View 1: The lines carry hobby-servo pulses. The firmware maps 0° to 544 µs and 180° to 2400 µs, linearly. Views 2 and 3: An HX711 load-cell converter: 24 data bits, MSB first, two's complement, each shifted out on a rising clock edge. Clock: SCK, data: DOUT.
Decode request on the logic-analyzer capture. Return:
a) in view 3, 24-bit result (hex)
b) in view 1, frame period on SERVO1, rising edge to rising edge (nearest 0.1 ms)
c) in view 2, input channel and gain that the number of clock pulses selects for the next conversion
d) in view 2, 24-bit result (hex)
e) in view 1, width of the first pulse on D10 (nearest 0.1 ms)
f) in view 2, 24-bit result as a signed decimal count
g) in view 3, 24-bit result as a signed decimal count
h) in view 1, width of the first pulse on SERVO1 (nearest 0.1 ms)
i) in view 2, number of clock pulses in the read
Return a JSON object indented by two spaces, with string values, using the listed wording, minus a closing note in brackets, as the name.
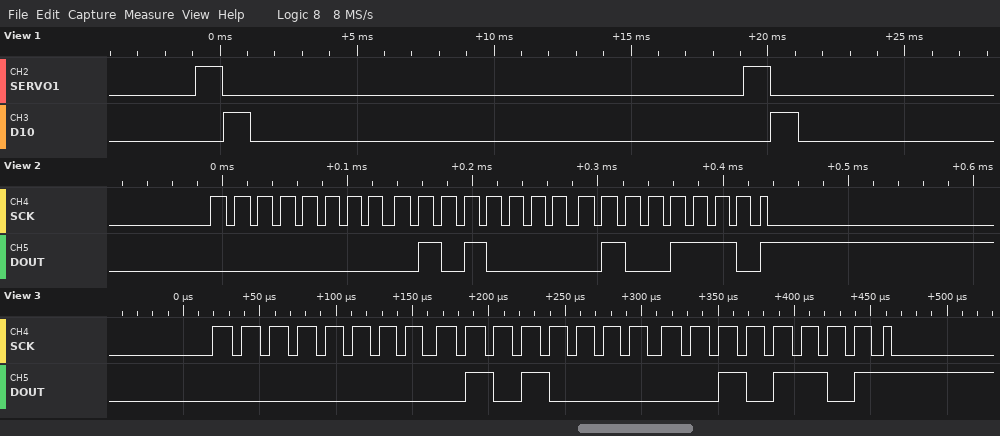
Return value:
{
  "in view 3, 24-bit result": "0x00502D",
  "in view 1, frame period on SERVO1, rising edge to rising edge": "20.0 ms",
  "in view 2, input channel and gain that the number of clock pulses selects for the next conversion": "channel A, gain 128",
  "in view 2, 24-bit result": "0x00504E",
  "in view 1, width of the first pulse on D10": "1.0 ms",
  "in view 2, 24-bit result as a signed decimal count": "20558",
  "in view 3, 24-bit result as a signed decimal count": "20525",
  "in view 1, width of the first pulse on SERVO1": "1.0 ms",
  "in view 2, number of clock pulses in the read": "25"
}
